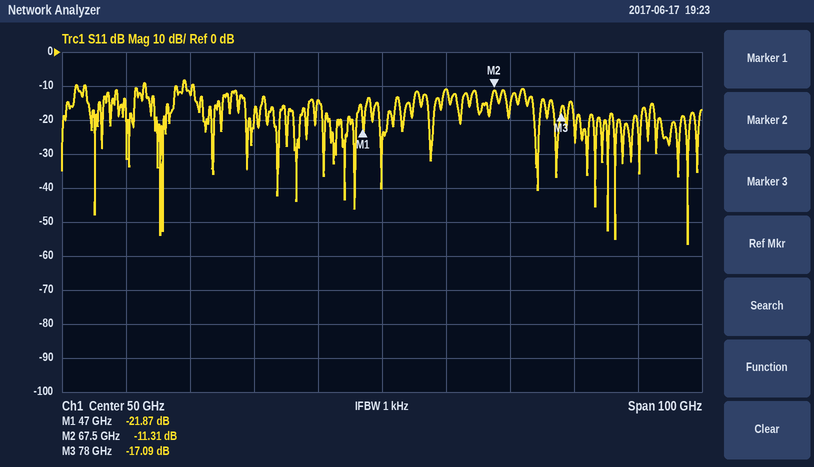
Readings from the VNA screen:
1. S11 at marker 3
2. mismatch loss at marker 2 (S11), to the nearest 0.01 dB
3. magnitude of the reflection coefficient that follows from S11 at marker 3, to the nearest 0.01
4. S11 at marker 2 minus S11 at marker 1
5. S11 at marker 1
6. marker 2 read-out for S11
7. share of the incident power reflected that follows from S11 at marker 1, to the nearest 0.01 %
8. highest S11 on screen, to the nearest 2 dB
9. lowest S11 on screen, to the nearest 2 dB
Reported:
-17.09 dB
0.33 dB
0.14
10.56 dB
-21.87 dB
-11.31 dB
0.65 %
-8 dB
-56 dB
